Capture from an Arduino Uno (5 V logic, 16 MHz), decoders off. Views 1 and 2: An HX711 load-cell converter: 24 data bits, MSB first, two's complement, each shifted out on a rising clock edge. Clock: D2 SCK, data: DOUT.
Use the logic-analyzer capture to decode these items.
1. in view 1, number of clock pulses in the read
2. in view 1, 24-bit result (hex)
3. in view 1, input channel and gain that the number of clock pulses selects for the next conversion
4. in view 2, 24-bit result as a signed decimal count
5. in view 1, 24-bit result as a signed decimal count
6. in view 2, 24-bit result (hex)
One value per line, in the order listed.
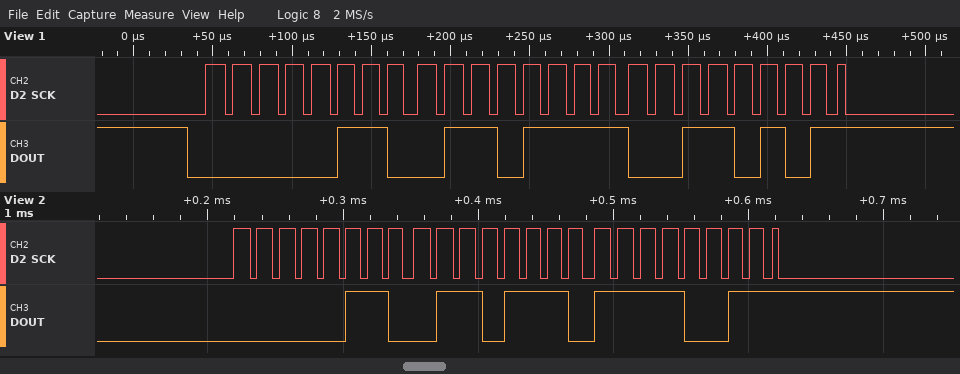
25
0x066F35
channel A, gain 128
421619
421685
0x066EF3
